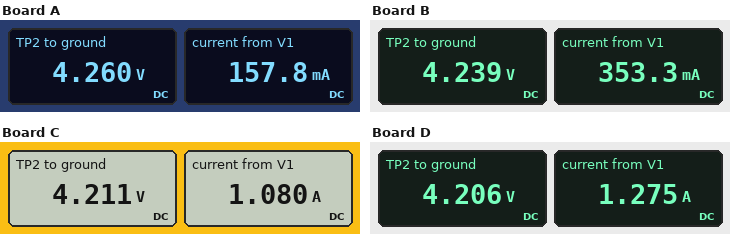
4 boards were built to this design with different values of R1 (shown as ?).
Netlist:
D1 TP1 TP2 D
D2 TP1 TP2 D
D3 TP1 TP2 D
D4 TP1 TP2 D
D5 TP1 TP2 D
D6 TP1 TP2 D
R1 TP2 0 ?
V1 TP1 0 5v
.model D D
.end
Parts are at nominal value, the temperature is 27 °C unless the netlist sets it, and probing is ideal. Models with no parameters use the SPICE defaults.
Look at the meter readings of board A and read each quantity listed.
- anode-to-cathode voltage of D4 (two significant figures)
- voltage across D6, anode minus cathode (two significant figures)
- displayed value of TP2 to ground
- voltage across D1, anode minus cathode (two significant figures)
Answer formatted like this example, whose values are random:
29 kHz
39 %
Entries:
740 mV
740 mV
4.260 V
740 mV
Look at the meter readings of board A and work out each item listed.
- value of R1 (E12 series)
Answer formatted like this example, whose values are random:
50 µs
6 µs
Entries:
27 Ω
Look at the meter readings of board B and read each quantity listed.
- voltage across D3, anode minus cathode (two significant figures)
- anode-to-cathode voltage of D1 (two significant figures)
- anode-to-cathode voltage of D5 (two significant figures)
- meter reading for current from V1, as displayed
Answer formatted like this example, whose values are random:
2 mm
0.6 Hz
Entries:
760 mV
760 mV
760 mV
353.3 mA
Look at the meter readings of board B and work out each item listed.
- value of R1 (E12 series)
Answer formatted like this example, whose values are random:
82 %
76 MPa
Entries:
12 Ω
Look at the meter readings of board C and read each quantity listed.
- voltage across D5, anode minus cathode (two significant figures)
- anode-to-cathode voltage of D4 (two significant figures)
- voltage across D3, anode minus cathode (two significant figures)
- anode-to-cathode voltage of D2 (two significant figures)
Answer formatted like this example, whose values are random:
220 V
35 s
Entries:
790 mV
790 mV
790 mV
790 mV
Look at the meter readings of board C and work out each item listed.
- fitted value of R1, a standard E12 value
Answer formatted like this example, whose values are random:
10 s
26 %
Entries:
3.9 Ω
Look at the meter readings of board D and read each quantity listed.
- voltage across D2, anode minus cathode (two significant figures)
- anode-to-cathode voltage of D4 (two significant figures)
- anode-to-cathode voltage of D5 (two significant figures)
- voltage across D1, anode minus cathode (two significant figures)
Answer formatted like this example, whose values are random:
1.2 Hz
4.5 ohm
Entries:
790 mV
790 mV
790 mV
790 mV
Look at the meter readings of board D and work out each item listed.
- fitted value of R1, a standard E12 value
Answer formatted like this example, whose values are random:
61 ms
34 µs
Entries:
3.3 Ω
